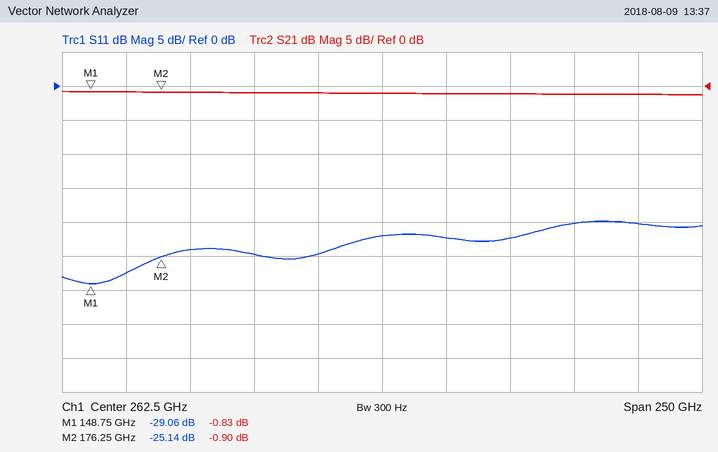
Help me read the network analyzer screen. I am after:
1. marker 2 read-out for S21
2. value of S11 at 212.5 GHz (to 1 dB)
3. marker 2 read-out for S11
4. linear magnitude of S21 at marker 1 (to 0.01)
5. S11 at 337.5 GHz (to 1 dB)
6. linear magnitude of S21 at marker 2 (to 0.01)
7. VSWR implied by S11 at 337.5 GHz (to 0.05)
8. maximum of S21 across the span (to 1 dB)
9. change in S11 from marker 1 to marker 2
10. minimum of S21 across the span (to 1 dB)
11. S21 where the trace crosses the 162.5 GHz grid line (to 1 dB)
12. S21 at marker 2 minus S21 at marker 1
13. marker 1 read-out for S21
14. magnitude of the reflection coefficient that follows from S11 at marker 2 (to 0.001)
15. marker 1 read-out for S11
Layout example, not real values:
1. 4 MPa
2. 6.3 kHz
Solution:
1. -0.90 dB
2. -25 dB
3. -25.14 dB
4. 0.91
5. -20 dB
6. 0.90
7. 1.20
8. -1 dB
9. 3.92 dB
10. -1 dB
11. -1 dB
12. -0.07 dB
13. -0.83 dB
14. 0.055
15. -29.06 dB
